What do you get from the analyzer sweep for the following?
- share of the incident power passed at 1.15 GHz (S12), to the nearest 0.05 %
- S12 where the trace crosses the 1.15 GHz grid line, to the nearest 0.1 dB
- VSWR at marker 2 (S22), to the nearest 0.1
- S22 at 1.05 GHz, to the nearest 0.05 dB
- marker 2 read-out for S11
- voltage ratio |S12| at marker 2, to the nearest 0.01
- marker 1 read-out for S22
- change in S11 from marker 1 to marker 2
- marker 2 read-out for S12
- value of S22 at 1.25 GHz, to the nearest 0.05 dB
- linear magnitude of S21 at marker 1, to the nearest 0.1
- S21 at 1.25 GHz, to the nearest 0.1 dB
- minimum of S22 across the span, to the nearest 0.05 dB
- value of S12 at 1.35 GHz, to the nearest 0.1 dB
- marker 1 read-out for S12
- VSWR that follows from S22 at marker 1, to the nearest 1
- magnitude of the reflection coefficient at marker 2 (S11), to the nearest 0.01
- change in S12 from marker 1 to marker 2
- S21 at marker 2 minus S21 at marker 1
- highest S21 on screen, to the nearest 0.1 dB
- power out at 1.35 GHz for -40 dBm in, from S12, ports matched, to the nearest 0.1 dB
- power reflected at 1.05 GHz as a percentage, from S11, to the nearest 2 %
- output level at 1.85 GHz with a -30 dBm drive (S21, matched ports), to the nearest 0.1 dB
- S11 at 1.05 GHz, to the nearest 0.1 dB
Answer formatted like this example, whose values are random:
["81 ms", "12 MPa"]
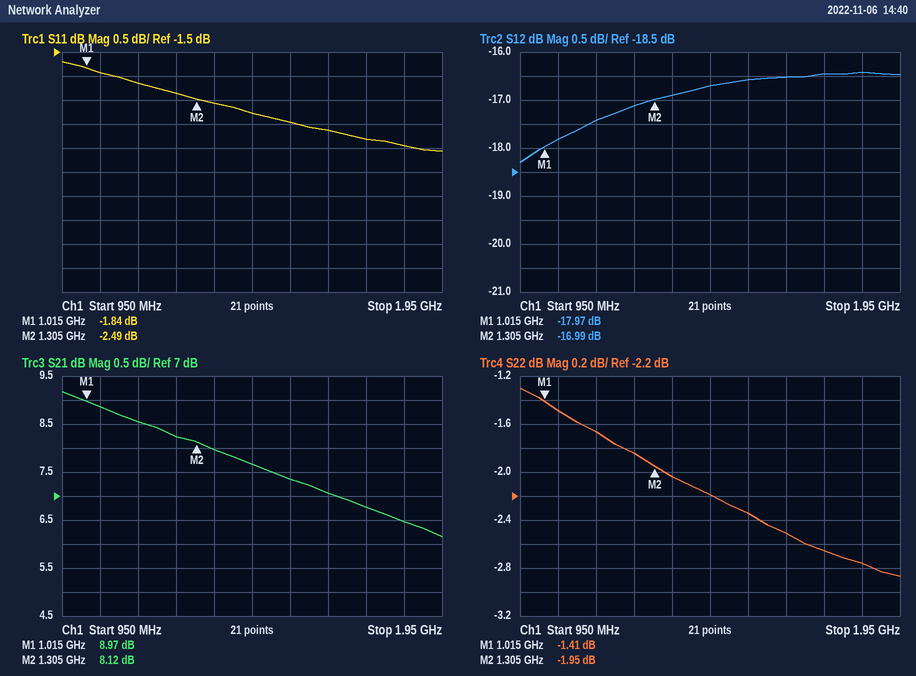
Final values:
["1.80 %", "-17.4 dB", "8.9", "-1.50 dB", "-2.49 dB", "0.14", "-1.41 dB", "-0.65 dB", "-16.99 dB", "-1.85 dB", "2.8", "8.2 dB", "-2.85 dB", "-16.9 dB", "-17.97 dB", "12", "0.75", "0.98 dB", "-0.85 dB", "9.2 dB", "-56.9 dBm", "64 %", "-23.5 dBm", "-1.9 dB"]
